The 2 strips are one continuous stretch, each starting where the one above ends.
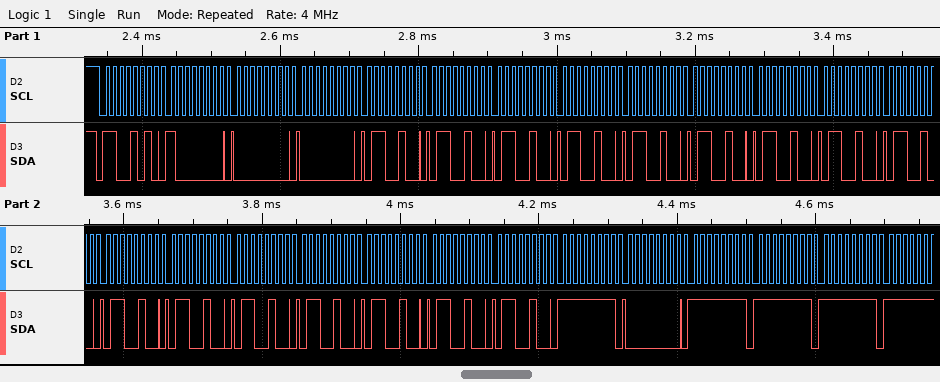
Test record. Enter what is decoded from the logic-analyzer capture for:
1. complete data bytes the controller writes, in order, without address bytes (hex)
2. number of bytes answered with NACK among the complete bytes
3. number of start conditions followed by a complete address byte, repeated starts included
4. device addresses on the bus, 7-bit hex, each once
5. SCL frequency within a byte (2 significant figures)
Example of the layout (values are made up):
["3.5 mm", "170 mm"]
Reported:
["80 00 00 64 64 64 64 64 64 64 64 64 64 64 64 64 64 64 64 FF 00 FF FF FF", "0", "1", "0x65", "100 kHz"]
